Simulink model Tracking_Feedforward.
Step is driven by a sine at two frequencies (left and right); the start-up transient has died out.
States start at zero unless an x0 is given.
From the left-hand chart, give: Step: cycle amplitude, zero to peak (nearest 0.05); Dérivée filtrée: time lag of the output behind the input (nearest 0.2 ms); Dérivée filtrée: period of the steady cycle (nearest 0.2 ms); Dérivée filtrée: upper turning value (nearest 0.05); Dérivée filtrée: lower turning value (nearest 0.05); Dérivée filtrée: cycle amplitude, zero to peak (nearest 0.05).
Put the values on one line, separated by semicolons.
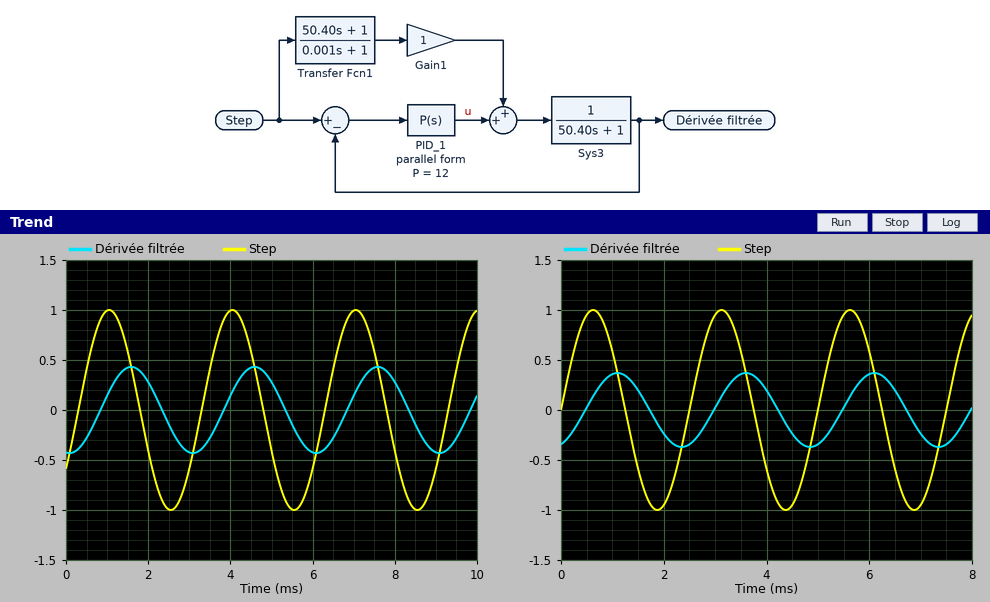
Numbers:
1.00; 0.6 ms; 3.0 ms; 0.45; -0.45; 0.45
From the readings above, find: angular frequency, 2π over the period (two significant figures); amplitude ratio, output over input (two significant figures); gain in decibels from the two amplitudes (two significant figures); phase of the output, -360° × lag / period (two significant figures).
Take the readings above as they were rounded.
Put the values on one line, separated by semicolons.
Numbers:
2.1 rad/ms; 0.45; -6.9 dB; -72°
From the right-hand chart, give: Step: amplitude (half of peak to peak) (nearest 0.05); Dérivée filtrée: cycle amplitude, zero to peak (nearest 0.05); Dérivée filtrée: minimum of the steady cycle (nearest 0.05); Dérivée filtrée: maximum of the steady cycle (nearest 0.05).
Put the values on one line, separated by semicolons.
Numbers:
1.00; 0.35; -0.35; 0.35
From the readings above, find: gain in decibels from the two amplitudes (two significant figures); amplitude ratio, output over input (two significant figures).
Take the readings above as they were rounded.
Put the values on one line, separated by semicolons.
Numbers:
-9.1 dB; 0.35
